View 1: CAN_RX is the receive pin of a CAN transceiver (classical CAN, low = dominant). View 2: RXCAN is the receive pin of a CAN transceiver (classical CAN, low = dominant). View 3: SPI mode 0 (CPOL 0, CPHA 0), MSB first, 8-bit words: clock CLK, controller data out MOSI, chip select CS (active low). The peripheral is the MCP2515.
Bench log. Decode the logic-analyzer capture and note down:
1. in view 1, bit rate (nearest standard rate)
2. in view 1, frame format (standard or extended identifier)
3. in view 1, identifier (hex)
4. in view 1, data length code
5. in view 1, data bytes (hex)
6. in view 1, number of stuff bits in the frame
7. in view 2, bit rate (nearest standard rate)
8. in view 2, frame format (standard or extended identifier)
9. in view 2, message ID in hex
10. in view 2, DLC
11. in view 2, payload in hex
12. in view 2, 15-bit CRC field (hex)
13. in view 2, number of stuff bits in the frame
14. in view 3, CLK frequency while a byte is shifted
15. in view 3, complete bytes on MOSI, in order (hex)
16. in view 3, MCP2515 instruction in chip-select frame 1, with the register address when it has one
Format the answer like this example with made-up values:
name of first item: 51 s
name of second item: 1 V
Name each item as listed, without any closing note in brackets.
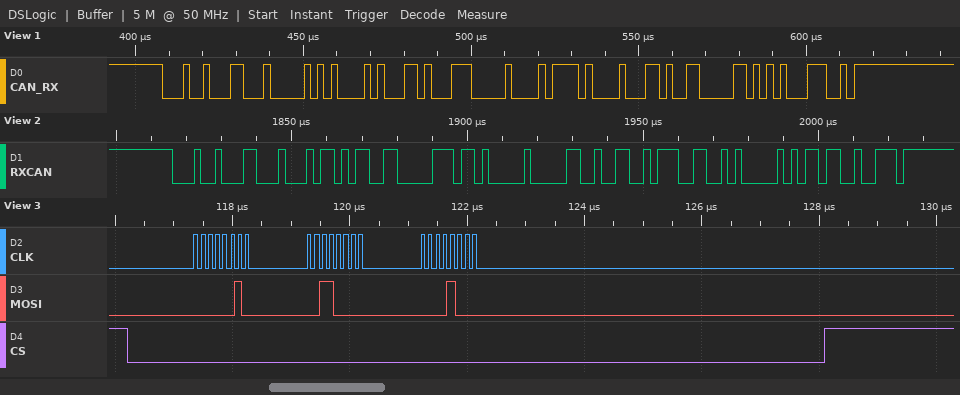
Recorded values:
in view 1, bit rate: 500 kbit/s
in view 1, frame format: standard
in view 1, identifier: 0x123
in view 1, data length code: 8
in view 1, data bytes: 14 28 D1 C0 17 A1 1A 60
in view 1, number of stuff bits in the frame: 3
in view 2, bit rate: 500 kbit/s
in view 2, frame format: standard
in view 2, message ID in hex: 0x123
in view 2, DLC: 8
in view 2, payload in hex: B5 98 36 80 12 65 CC A0
in view 2, 15-bit CRC field: 0x2D93
in view 2, number of stuff bits in the frame: 4
in view 3, CLK frequency while a byte is shifted: 8 MHz
in view 3, complete bytes on MOSI, in order: 02 30 08
in view 3, MCP2515 instruction in chip-select frame 1, with the register address when it has one: WRITE 0x30
